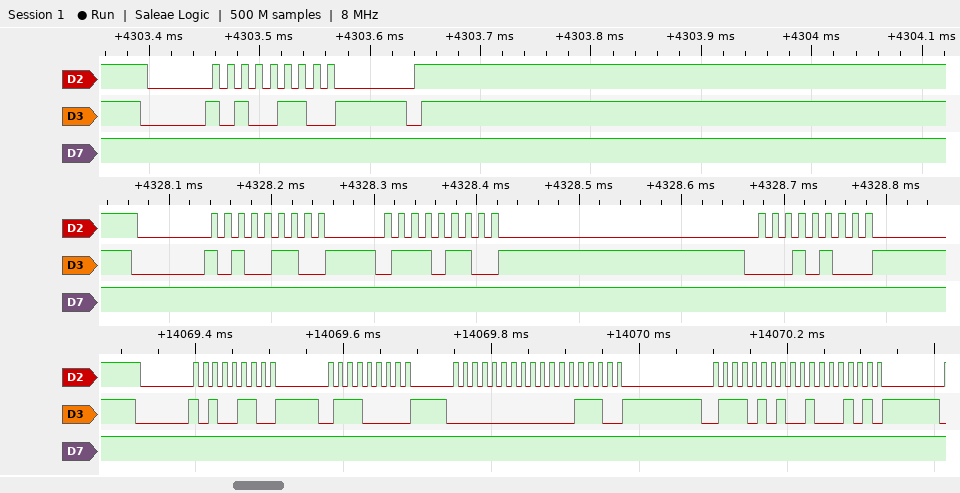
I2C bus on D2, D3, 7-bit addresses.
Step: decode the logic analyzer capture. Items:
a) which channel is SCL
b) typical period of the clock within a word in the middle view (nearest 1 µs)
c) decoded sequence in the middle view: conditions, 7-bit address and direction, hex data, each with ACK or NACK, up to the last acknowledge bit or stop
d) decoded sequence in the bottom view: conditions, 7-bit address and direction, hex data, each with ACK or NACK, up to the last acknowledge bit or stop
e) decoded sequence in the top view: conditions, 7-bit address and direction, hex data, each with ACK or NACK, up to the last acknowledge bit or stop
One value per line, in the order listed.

D2
13 µs
start, address 53 write ACK, 76 ACK, 14 ACK
start, address 53 write ACK, 70 ACK, 00 ACK, 0E ACK, 75 ACK, 45 ACK
start, address 53 write ACK, stop
